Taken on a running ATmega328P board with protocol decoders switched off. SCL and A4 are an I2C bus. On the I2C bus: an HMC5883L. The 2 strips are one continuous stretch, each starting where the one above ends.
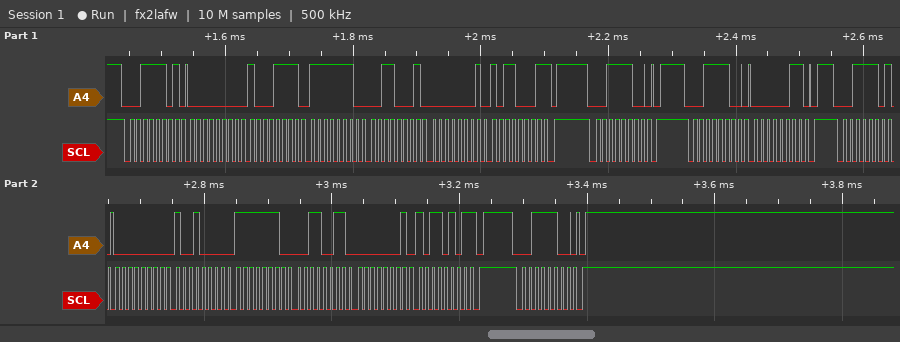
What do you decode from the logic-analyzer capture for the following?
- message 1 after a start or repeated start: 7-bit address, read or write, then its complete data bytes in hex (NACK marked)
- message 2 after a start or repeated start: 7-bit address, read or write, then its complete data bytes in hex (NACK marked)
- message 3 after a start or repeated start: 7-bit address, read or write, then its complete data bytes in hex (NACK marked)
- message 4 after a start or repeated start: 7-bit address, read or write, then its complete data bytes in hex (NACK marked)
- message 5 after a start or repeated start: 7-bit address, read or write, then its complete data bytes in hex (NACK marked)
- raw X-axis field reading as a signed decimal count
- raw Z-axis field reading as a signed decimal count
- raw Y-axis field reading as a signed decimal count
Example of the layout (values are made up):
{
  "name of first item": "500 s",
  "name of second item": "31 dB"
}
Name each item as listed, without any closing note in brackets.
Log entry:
{
  "message 1 after a start or repeated start: 7-bit address, read or write, then its complete data bytes in hex": "0x1E read: 00 8F FE 31 01 B1 NACK",
  "message 2 after a start or repeated start: 7-bit address, read or write, then its complete data bytes in hex": "0x1E write",
  "message 3 after a start or repeated start: 7-bit address, read or write, then its complete data bytes in hex": "0x1E write: 03",
  "message 4 after a start or repeated start: 7-bit address, read or write, then its complete data bytes in hex": "0x1E read: 00 90 FE 33 01 B5 NACK",
  "message 5 after a start or repeated start: 7-bit address, read or write, then its complete data bytes in hex": "0x1E write",
  "raw X-axis field reading as a signed decimal count": "144",
  "raw Z-axis field reading as a signed decimal count": "-461",
  "raw Y-axis field reading as a signed decimal count": "437"
}
